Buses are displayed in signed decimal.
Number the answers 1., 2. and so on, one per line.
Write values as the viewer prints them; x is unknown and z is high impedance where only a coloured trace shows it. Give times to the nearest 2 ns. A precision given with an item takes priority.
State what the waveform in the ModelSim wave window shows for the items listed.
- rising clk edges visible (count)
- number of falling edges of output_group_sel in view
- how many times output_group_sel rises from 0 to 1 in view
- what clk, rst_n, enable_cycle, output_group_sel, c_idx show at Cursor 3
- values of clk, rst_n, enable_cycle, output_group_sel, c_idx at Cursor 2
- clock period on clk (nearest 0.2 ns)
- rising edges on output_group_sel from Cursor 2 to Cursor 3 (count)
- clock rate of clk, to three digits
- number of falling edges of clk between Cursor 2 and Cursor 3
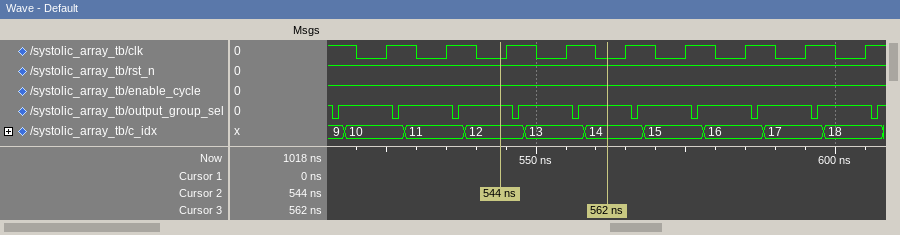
1. 9
2. 10
3. 10
4. clk=0, rst_n=1, enable_cycle=1, output_group_sel=1, c_idx=14
5. clk=0, rst_n=1, enable_cycle=1, output_group_sel=1, c_idx=12
6. 10 ns
7. 2
8. 100 MHz
9. 2
